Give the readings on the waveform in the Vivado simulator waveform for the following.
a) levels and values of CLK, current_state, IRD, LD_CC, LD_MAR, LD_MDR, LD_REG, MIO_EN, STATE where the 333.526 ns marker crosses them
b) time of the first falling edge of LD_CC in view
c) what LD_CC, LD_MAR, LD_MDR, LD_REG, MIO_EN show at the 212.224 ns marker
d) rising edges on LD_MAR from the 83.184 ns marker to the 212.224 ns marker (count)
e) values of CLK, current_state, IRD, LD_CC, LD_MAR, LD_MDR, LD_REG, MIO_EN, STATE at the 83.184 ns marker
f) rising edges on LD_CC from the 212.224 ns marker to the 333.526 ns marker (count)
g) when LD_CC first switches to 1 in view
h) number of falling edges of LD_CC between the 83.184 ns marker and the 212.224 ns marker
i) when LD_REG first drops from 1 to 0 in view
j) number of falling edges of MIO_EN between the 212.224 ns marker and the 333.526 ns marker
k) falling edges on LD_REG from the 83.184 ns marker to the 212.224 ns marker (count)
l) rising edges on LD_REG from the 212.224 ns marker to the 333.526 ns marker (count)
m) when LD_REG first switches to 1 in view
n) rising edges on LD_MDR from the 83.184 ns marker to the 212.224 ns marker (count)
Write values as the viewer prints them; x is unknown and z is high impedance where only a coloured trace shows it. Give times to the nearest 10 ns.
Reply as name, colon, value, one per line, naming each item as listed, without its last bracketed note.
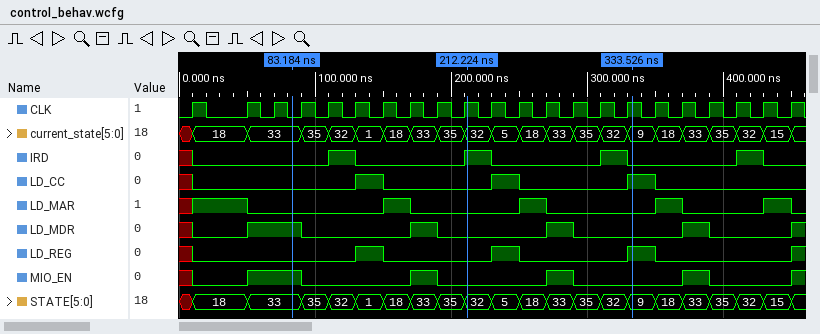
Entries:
levels and values of CLK, current_state, IRD, LD_CC, LD_MAR, LD_MDR, LD_REG, MIO_EN, STATE where the 333.526 ns marker crosses them: CLK=1, current_state=9, IRD=0, LD_CC=1, LD_MAR=0, LD_MDR=0, LD_REG=1, MIO_EN=0, STATE=9
time of the first falling edge of LD_CC in view: 150 ns
what LD_CC, LD_MAR, LD_MDR, LD_REG, MIO_EN show at the 212.224 ns marker: LD_CC=0, LD_MAR=0, LD_MDR=0, LD_REG=0, MIO_EN=0
rising edges on LD_MAR from the 83.184 ns marker to the 212.224 ns marker: 1
values of CLK, current_state, IRD, LD_CC, LD_MAR, LD_MDR, LD_REG, MIO_EN, STATE at the 83.184 ns marker: CLK=0, current_state=33, IRD=0, LD_CC=0, LD_MAR=0, LD_MDR=1, LD_REG=0, MIO_EN=1, STATE=33
rising edges on LD_CC from the 212.224 ns marker to the 333.526 ns marker: 2
when LD_CC first switches to 1 in view: 130 ns
number of falling edges of LD_CC between the 83.184 ns marker and the 212.224 ns marker: 1
when LD_REG first drops from 1 to 0 in view: 150 ns
number of falling edges of MIO_EN between the 212.224 ns marker and the 333.526 ns marker: 1
falling edges on LD_REG from the 83.184 ns marker to the 212.224 ns marker: 1
rising edges on LD_REG from the 212.224 ns marker to the 333.526 ns marker: 2
when LD_REG first switches to 1 in view: 130 ns
rising edges on LD_MDR from the 83.184 ns marker to the 212.224 ns marker: 1
